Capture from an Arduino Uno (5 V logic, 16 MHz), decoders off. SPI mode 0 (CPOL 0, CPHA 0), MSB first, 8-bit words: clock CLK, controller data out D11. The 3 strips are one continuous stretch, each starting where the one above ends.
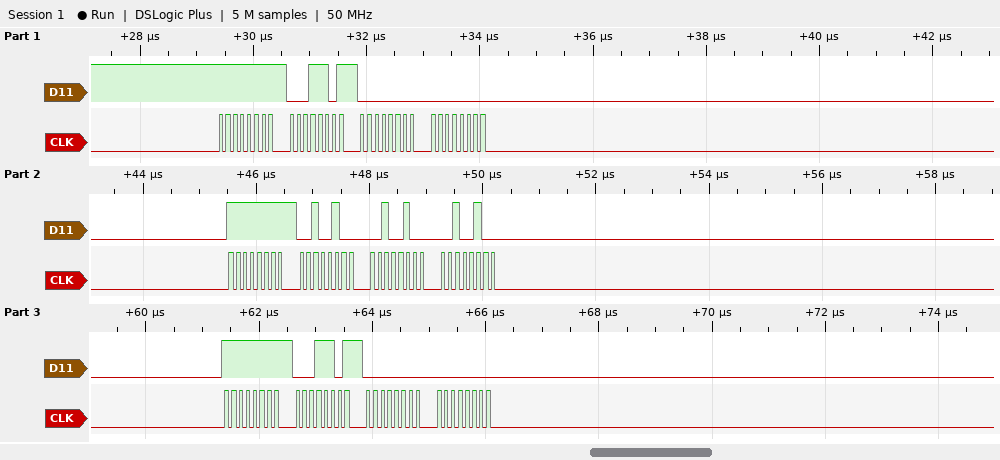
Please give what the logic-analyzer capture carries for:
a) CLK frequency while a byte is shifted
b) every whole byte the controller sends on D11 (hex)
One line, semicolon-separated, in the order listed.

8 MHz; FF 1D 00 00 FF 24 24 24 FF 1D 00 00
